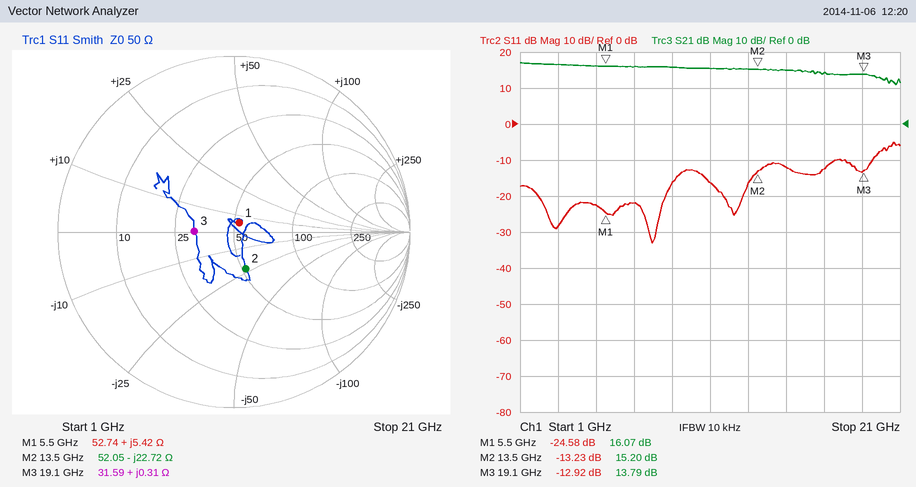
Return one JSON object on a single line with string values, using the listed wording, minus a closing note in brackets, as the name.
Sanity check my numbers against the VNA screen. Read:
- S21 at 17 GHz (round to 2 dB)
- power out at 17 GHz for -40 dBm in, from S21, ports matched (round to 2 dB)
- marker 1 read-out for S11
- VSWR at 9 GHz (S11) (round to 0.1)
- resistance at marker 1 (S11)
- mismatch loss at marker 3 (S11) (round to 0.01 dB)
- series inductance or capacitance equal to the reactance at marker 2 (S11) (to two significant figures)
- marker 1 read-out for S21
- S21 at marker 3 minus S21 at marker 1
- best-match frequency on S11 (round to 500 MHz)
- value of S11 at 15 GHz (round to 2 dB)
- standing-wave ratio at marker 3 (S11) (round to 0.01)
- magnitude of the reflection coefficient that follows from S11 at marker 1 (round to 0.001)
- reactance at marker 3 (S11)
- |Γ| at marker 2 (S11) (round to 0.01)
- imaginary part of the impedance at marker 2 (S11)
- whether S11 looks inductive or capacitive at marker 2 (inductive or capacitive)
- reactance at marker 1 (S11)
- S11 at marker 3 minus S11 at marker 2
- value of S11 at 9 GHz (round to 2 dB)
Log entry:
{"S21 at 17 GHz": "14 dB", "power out at 17 GHz for -40 dBm in, from S21, ports matched": "-26 dBm", "marker 1 read-out for S11": "-24.58 dB", "VSWR at 9 GHz (S11)": "1.4", "resistance at marker 1": "52.74 Ω", "mismatch loss at marker 3 (S11)": "0.23 dB", "series inductance or capacitance equal to the reactance at marker 2 (S11)": "520 fF", "marker 1 read-out for S21": "16.07 dB", "S21 at marker 3 minus S21 at marker 1": "-2.28 dB", "best-match frequency on S11": "8.0 GHz", "value of S11 at 15 GHz": "-12 dB", "standing-wave ratio at marker 3 (S11)": "1.58", "magnitude of the reflection coefficient that follows from S11 at marker 1": "0.059", "reactance at marker 3": "+0.31 Ω", "|Γ| at marker 2 (S11)": "0.22", "imaginary part of the impedance at marker 2": "-22.72 Ω", "whether S11 looks inductive or capacitive at marker 2": "capacitive", "reactance at marker 1": "+5.42 Ω", "S11 at marker 3 minus S11 at marker 2": "0.31 dB", "value of S11 at 9 GHz": "-16 dB"}
